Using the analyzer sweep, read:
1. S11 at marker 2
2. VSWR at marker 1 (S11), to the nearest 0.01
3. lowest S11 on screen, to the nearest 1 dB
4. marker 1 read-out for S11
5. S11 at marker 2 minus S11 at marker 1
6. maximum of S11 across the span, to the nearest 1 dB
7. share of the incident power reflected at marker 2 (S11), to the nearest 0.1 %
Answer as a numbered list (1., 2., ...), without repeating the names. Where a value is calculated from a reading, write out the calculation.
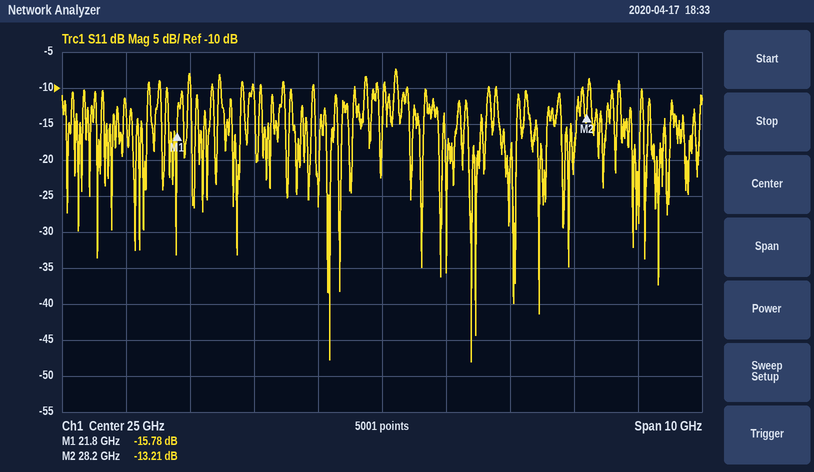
1. -13.21 dB
2. (1 + 0.1626)/(1 − 0.1626) ≈ 1.39
3. -48 dB
4. -15.78 dB
5. -13.21 − (-15.78) = 2.57 dB
6. -7 dB
7. 10^(-13.21/10) ≈ 4.8 %
